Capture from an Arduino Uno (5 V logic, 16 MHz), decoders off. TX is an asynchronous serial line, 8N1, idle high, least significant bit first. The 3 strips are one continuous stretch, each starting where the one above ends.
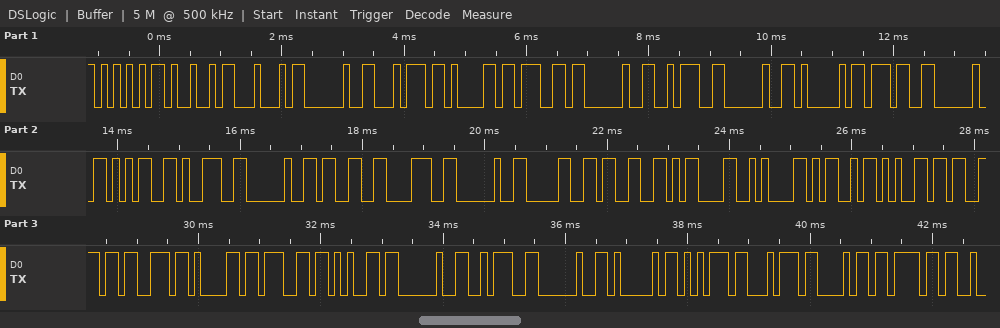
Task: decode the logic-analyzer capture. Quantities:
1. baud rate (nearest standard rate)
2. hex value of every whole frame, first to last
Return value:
9600 baud
0x55 0x49 0x44 0x20 0x74 0x61 0x67 0x20 0x3A 0x20 0x41 0x37 0x20 0x35 0x39 0x20 0x33 0x38 0x20 0x30 0x33 0x0D 0x0A 0x4D 0x65 0x73 0x73 0x61 0x67 0x65 0x20 0x3A 0x20 0x41 0x75 0x74 0x68 0x6F
